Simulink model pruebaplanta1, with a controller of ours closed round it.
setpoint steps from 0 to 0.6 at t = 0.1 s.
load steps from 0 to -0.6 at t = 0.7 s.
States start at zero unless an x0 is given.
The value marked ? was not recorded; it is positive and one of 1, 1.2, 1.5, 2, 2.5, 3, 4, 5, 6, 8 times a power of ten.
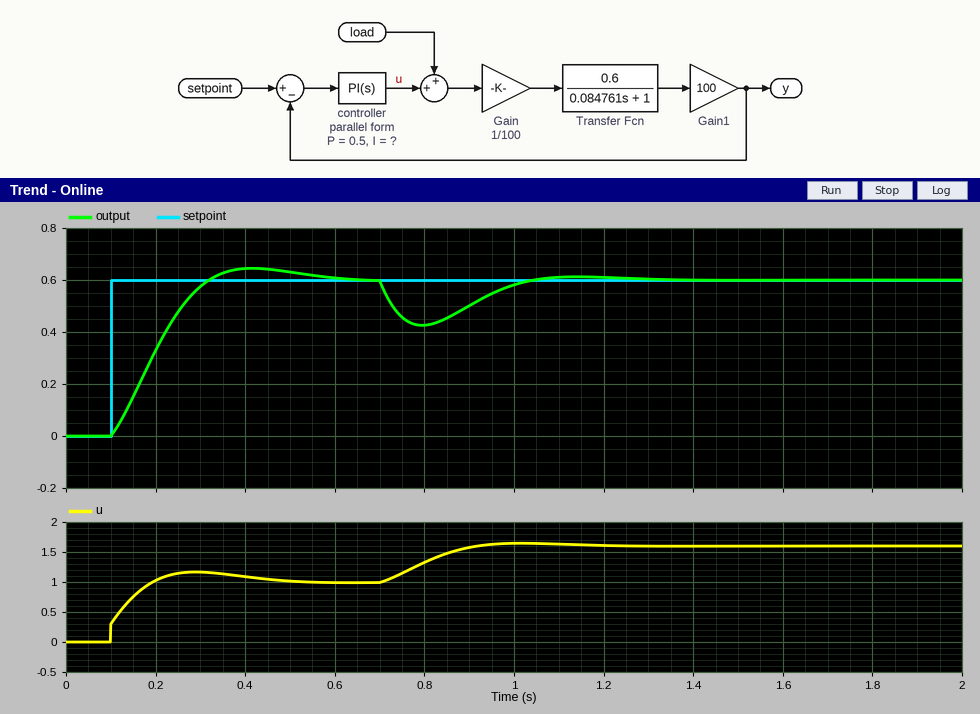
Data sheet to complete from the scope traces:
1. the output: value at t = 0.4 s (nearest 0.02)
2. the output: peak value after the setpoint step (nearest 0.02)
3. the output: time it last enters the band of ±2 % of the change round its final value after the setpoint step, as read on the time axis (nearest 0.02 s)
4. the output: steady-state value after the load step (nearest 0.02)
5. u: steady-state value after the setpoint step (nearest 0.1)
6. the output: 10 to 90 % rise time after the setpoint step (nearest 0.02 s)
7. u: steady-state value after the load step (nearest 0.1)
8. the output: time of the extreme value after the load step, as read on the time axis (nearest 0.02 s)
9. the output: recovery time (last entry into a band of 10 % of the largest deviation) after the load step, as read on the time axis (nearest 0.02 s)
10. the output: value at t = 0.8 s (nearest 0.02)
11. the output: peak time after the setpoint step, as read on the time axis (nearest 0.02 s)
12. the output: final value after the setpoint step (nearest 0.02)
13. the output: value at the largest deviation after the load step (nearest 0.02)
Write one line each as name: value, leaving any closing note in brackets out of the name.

the output: value at t = 0.4 s: 0.64
the output: peak value after the setpoint step: 0.64
the output: time it last enters the band of ±2 % of the change round its final value after the setpoint step, as read on the time axis: 0.58 s
the output: steady-state value after the load step: 0.60
u: steady-state value after the setpoint step: 1.0
the output: 10 to 90 % rise time after the setpoint step: 0.16 s
u: steady-state value after the load step: 1.6
the output: time of the extreme value after the load step, as read on the time axis: 0.80 s
the output: recovery time (last entry into a band of 10 % of the largest deviation) after the load step, as read on the time axis: 1.00 s
the output: value at t = 0.8 s: 0.42
the output: peak time after the setpoint step, as read on the time axis: 0.42 s
the output: final value after the setpoint step: 0.60
the output: value at the largest deviation after the load step: 0.42
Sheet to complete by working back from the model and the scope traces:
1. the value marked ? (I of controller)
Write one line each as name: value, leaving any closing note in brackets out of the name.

the value marked ?: 20
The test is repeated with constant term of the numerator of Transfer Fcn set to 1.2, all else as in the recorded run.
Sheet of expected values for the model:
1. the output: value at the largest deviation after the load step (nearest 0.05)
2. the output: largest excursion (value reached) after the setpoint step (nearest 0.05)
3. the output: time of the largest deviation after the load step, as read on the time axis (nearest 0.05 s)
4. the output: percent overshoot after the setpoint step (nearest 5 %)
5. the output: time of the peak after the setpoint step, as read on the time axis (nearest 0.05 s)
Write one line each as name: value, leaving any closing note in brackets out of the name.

the output: value at the largest deviation after the load step: 0.35
the output: largest excursion (value reached) after the setpoint step: 0.70
the output: time of the largest deviation after the load step, as read on the time axis: 0.75 s
the output: percent overshoot after the setpoint step: 15 %
the output: time of the peak after the setpoint step, as read on the time axis: 0.30 s
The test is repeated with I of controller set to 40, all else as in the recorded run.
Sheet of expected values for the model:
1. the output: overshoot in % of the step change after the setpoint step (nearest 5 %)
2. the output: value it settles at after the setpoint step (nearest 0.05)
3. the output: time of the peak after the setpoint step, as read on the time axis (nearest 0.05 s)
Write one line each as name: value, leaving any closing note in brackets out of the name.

the output: overshoot in % of the step change after the setpoint step: 20 %
the output: value it settles at after the setpoint step: 0.60
the output: time of the peak after the setpoint step, as read on the time axis: 0.30 s
